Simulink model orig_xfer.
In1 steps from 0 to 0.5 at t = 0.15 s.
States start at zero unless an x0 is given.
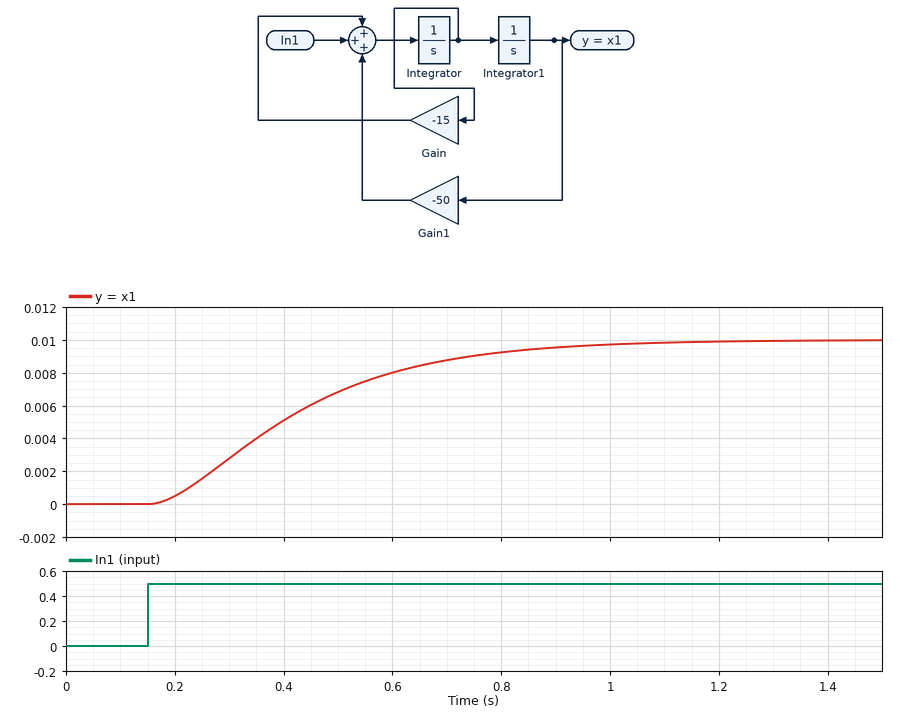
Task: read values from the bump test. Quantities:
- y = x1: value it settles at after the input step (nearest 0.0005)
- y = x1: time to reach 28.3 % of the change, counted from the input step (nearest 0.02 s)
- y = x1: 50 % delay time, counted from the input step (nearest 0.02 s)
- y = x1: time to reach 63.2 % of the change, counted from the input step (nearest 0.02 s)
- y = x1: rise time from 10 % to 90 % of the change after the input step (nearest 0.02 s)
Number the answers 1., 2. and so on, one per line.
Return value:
1. 0.0100
2. 0.16 s
3. 0.24 s
4. 0.32 s
5. 0.52 s
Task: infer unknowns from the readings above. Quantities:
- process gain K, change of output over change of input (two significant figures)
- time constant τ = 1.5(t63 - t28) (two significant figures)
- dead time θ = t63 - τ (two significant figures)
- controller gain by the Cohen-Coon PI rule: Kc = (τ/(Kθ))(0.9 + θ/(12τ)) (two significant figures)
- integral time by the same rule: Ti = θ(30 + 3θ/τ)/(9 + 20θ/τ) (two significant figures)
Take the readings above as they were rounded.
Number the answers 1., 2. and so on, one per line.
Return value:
1. 0.020
2. 0.24 s
3. 0.080 s
4. 140
5. 0.16 s
